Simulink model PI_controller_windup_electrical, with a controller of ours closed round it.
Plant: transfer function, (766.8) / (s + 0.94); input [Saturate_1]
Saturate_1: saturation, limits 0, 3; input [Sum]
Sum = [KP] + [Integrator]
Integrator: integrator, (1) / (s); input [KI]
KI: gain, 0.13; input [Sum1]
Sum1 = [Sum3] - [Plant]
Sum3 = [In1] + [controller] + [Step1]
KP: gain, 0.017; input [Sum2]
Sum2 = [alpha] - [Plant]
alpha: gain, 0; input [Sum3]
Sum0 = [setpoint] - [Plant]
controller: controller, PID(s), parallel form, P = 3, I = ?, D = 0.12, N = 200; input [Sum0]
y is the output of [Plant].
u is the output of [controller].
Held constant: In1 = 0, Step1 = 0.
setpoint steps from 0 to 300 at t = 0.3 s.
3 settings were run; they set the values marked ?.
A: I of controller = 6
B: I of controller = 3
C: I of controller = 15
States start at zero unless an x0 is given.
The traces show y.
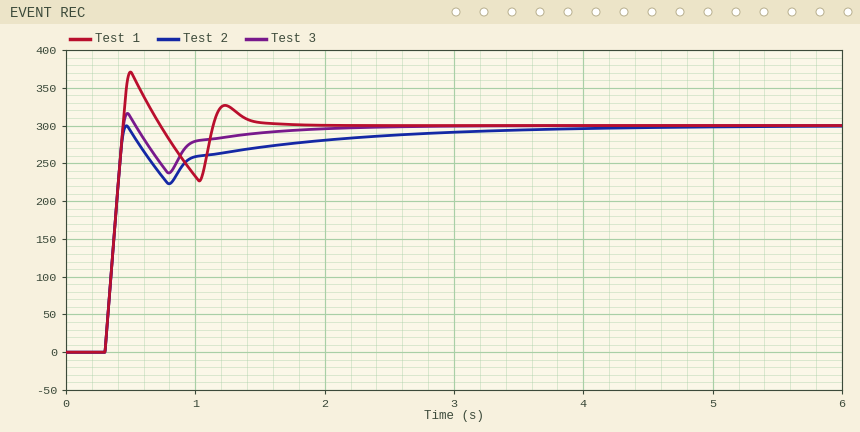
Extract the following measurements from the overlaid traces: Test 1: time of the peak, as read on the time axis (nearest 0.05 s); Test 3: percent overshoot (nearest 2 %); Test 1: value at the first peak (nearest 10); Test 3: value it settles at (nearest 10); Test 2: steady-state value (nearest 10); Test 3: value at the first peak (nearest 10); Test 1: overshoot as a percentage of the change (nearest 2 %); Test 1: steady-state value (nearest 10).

0.50 s
6 %
370
300
300
320
24 %
300
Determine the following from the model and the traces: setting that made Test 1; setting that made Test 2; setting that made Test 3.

C
B
A
